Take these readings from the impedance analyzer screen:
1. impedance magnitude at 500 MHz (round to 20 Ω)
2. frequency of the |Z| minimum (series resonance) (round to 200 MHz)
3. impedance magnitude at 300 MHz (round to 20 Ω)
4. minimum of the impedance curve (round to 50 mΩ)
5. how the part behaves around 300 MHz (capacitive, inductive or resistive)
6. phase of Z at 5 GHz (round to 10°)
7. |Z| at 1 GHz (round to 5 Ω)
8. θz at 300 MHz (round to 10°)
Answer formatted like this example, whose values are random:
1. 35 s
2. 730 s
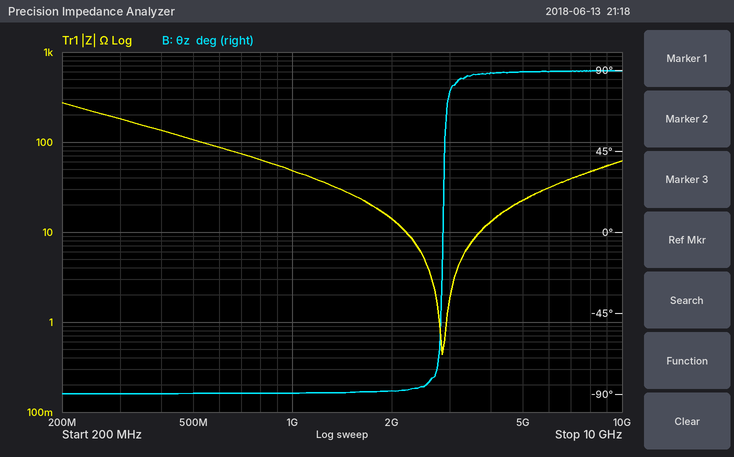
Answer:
1. 100 Ω
2. 2.8 GHz
3. 180 Ω
4. 450 mΩ
5. capacitive
6. 90°
7. 50 Ω
8. -90°
